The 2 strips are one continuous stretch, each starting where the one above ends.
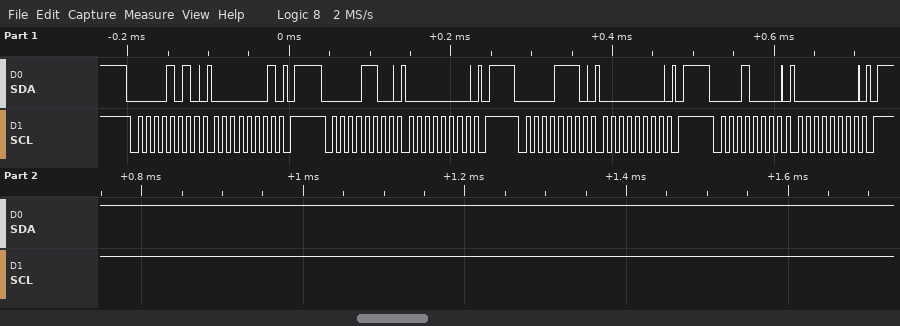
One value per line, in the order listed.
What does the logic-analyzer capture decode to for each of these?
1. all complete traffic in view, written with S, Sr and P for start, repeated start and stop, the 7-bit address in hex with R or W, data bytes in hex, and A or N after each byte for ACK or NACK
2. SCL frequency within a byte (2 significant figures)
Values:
S 05W A 01 A P S 06W A 00 A P S 07W A 00 A P S 08W A 00 A P
100 kHz
